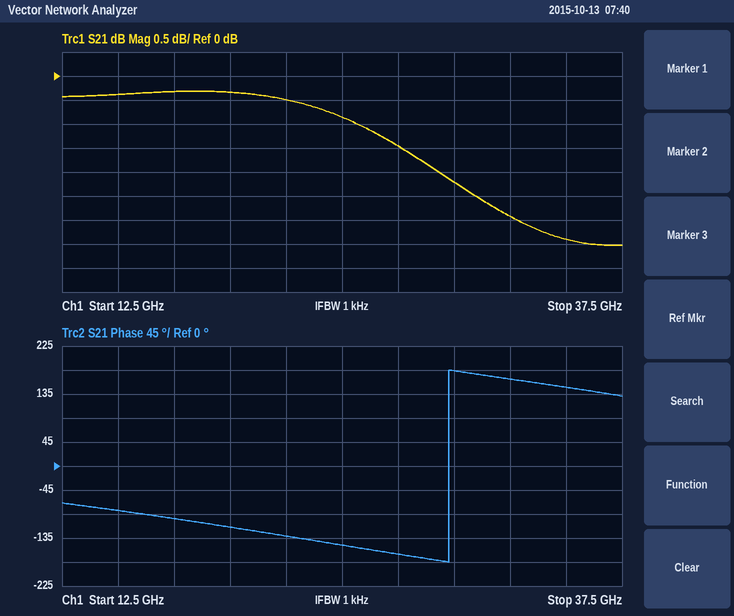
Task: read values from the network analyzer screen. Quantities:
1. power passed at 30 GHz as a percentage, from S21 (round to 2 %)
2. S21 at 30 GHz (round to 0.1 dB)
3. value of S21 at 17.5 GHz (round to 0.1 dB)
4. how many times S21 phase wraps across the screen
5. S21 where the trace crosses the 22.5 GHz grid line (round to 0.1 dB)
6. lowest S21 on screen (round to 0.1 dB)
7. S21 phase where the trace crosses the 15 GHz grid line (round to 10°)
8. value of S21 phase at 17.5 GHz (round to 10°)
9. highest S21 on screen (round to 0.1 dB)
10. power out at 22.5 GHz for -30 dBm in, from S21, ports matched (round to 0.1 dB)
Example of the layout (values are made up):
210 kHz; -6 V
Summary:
60 %; -2.2 dB; -0.3 dB; 1; -0.5 dB; -3.5 dB; -80°; -100°; -0.3 dB; -30.5 dBm
